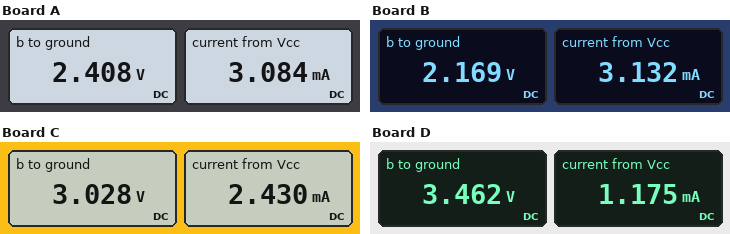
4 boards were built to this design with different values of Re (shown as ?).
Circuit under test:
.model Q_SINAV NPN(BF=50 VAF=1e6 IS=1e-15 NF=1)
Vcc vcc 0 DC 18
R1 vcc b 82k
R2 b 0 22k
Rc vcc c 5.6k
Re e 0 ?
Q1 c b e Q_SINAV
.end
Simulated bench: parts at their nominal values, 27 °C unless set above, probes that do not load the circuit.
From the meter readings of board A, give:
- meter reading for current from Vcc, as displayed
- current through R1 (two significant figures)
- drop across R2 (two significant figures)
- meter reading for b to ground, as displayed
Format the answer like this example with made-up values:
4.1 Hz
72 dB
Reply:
3.084 mA
190 µA
2.4 V
2.408 V
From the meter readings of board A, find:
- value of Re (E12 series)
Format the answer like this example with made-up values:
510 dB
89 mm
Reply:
560 Ω
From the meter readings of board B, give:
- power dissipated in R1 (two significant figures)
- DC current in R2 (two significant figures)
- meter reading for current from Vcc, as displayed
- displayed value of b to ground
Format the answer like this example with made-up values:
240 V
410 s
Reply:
3.1 mW
99 µA
3.132 mA
2.169 V
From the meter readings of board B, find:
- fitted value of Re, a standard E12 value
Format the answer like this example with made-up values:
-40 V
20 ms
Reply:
470 Ω
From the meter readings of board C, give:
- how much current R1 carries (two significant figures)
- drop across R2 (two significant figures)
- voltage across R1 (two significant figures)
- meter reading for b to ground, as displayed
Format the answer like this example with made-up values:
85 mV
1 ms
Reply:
180 µA
3.0 V
15 V
3.028 V
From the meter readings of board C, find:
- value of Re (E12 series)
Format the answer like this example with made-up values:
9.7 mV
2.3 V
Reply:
1 kΩ
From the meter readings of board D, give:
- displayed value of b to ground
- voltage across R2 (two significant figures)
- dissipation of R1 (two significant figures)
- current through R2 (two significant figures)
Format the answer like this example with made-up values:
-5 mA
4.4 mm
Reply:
3.462 V
3.5 V
2.6 mW
160 µA
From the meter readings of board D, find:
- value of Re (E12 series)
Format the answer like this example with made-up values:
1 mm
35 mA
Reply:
2.7 kΩ
